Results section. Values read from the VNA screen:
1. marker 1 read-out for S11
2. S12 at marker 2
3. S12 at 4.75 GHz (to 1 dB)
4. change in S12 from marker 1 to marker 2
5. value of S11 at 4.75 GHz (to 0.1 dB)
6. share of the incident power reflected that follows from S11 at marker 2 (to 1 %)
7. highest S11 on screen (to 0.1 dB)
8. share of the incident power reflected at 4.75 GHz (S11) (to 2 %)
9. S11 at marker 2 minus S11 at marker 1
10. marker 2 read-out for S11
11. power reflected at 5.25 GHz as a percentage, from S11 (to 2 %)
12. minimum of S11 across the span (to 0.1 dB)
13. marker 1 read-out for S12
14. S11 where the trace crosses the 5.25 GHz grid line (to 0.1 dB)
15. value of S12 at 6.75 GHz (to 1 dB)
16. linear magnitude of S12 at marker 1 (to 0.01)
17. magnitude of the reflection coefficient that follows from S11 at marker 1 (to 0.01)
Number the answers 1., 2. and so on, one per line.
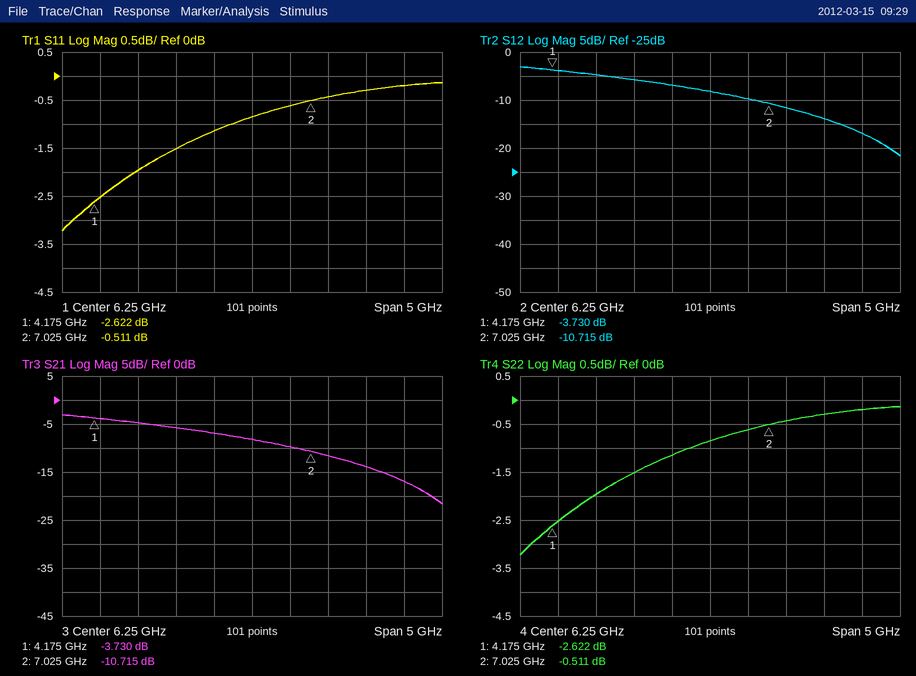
1. -2.622 dB
2. -10.715 dB
3. -5 dB
4. -6.985 dB
5. -2.0 dB
6. 89 %
7. -0.1 dB
8. 64 %
9. 2.111 dB
10. -0.511 dB
11. 70 %
12. -3.2 dB
13. -3.730 dB
14. -1.5 dB
15. -10 dB
16. 0.65
17. 0.74
